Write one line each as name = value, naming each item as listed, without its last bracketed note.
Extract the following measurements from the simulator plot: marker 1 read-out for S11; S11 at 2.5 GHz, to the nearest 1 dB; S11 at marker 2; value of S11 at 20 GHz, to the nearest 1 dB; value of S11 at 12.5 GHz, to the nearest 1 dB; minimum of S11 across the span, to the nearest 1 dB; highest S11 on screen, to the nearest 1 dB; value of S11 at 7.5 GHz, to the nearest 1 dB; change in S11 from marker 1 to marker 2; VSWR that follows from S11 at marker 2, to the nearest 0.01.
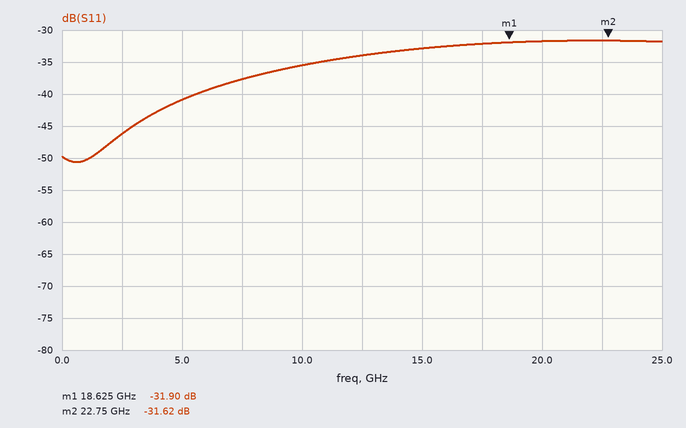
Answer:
marker 1 read-out for S11 = -31.90 dB
S11 at 2.5 GHz, to the nearest 1 dB = -46 dB
S11 at marker 2 = -31.62 dB
value of S11 at 20 GHz, to the nearest 1 dB = -32 dB
value of S11 at 12.5 GHz, to the nearest 1 dB = -34 dB
minimum of S11 across the span, to the nearest 1 dB = -51 dB
highest S11 on screen, to the nearest 1 dB = -32 dB
value of S11 at 7.5 GHz, to the nearest 1 dB = -38 dB
change in S11 from marker 1 to marker 2 = 0.28 dB
VSWR that follows from S11 at marker 2, to the nearest 0.01 = 1.05
